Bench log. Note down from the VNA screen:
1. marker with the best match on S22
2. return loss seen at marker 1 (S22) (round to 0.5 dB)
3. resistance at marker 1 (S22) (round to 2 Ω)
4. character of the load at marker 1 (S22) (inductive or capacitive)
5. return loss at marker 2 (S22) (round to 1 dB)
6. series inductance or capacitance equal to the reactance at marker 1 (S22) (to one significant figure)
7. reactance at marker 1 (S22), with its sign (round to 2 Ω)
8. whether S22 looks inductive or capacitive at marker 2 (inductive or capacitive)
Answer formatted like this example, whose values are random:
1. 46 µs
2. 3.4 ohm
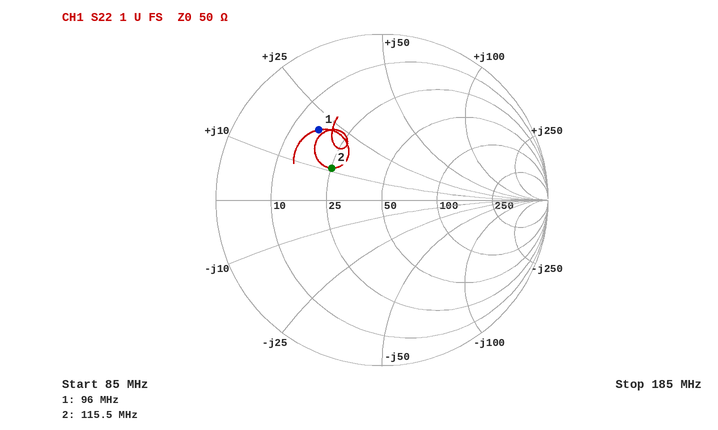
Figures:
1. marker 2
2. 5.0 dB
3. 16 Ω
4. inductive
5. 9 dB
6. 30 nH
7. +20 Ω
8. inductive
